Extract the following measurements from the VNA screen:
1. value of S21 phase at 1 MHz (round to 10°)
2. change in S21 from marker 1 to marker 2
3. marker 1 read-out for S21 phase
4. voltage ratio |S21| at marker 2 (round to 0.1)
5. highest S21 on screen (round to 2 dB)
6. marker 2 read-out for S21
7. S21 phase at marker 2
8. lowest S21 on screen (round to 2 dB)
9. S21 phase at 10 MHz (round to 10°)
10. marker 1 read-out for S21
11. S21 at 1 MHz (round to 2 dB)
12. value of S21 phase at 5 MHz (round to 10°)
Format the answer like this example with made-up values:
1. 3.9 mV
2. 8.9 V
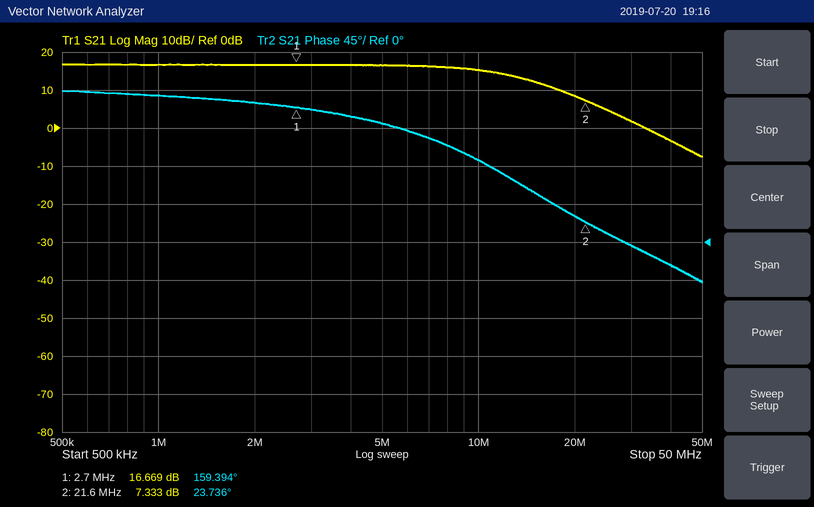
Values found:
1. 170°
2. -9.336 dB
3. 159.394°
4. 2.3
5. 16 dB
6. 7.333 dB
7. 23.736°
8. -8 dB
9. 100°
10. 16.669 dB
11. 16 dB
12. 140°
